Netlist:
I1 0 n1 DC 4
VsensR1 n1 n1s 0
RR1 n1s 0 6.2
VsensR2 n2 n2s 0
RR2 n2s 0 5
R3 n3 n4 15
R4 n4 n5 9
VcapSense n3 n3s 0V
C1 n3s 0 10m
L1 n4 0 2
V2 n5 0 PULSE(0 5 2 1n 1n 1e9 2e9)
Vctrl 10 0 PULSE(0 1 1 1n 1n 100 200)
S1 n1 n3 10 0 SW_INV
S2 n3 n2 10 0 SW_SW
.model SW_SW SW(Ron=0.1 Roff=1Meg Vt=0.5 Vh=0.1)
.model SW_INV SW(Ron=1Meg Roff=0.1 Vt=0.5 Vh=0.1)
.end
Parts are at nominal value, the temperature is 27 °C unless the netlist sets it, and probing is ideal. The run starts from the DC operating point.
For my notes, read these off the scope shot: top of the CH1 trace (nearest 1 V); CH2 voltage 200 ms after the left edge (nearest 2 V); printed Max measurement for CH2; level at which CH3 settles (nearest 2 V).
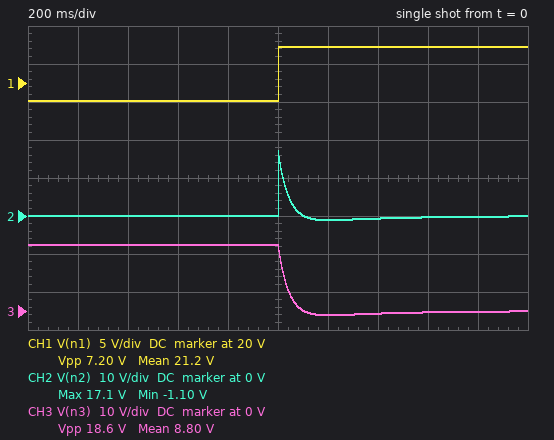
25 V
0 V
17.1 V
0 V
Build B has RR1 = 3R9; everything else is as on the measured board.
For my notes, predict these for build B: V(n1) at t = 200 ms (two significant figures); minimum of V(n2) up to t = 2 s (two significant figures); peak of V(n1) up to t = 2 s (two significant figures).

12 V
-770 mV
16 V
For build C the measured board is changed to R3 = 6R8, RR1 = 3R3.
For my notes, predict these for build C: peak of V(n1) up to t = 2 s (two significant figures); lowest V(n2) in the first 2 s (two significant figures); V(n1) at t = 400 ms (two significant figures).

13 V
-2.1 V
8.9 V
